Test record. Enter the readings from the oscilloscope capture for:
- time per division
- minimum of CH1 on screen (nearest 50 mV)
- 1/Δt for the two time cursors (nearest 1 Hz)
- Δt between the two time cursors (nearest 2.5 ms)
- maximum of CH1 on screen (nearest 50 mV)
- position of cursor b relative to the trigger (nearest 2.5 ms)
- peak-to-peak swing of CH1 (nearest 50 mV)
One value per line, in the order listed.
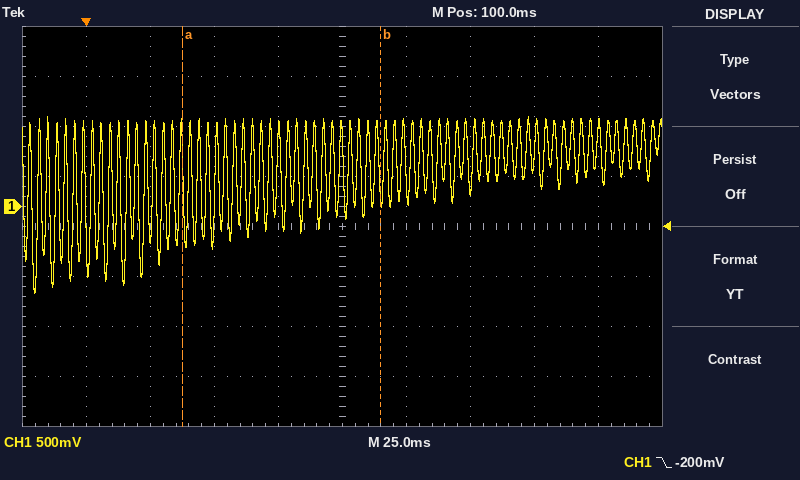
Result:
25 ms
-850 mV
13 Hz
77.5 ms
900 mV
+115.0 ms
1.75 V
